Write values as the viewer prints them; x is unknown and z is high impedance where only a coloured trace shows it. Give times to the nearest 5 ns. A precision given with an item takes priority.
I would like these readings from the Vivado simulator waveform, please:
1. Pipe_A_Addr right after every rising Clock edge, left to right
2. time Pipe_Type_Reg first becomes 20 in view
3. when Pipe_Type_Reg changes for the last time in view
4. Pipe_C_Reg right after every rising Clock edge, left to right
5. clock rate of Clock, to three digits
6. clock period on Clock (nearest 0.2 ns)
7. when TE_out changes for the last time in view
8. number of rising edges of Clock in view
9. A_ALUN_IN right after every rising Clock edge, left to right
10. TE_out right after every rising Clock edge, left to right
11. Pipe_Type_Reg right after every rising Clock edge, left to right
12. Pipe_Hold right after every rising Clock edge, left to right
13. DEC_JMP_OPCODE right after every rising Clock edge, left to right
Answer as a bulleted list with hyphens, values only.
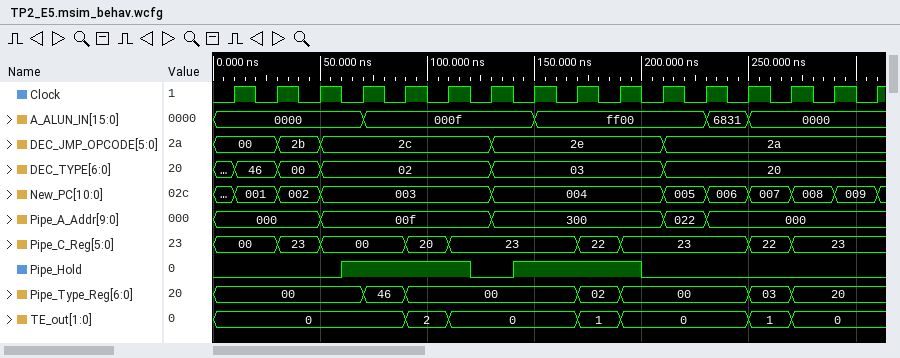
- 000, 000, 00f, 00f, 00f, 00f, 300, 300, 300, 300, 022, 000, 000, 000, 000, 000
- 270 ns
- 270 ns
- 00, 23, 00, 00, 20, 23, 23, 23, 22, 23, 23, 23, 22, 23, 23, 23
- 50.0 MHz
- 20 ns
- 270 ns
- 16
- 0000, 0000, 0000, 000f, 000f, 000f, 000f, ff00, ff00, ff00, ff00, 6831, 0000, 0000, 0000, 0000
- 0, 0, 0, 0, 2, 0, 0, 0, 1, 0, 0, 0, 1, 0, 0, 0
- 00, 00, 00, 46, 00, 00, 00, 00, 02, 00, 00, 00, 03, 20, 20, 20
- 0 0 0 1 1 1 0 1 1 1 0 0 0 0 0 0
- 00, 2b, 2c, 2c, 2c, 2c, 2e, 2e, 2e, 2e, 2a, 2a, 2a, 2a, 2a, 2a
